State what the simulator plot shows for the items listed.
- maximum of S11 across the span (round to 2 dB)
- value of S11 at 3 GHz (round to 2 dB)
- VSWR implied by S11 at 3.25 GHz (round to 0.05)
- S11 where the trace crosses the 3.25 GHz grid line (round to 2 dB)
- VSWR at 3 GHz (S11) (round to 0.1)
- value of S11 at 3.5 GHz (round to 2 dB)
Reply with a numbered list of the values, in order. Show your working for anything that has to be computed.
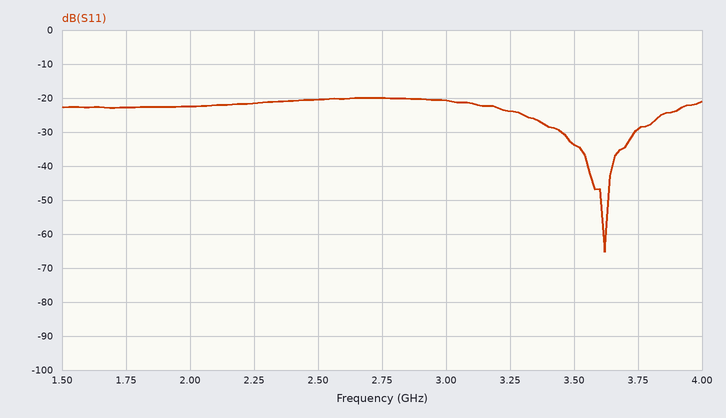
1. -20 dB
2. -20 dB
3. |Γ| = 10^(-24/20) = 0.0631; VSWR = (1 + 0.0631)/(1 − 0.0631) ≈ 1.13, so 1.15 to the nearest 0.05
4. -24 dB
5. |Γ| = 10^(-20/20) = 0.1000; VSWR = (1 + 0.1000)/(1 − 0.1000) ≈ 1.2
6. -34 dB
